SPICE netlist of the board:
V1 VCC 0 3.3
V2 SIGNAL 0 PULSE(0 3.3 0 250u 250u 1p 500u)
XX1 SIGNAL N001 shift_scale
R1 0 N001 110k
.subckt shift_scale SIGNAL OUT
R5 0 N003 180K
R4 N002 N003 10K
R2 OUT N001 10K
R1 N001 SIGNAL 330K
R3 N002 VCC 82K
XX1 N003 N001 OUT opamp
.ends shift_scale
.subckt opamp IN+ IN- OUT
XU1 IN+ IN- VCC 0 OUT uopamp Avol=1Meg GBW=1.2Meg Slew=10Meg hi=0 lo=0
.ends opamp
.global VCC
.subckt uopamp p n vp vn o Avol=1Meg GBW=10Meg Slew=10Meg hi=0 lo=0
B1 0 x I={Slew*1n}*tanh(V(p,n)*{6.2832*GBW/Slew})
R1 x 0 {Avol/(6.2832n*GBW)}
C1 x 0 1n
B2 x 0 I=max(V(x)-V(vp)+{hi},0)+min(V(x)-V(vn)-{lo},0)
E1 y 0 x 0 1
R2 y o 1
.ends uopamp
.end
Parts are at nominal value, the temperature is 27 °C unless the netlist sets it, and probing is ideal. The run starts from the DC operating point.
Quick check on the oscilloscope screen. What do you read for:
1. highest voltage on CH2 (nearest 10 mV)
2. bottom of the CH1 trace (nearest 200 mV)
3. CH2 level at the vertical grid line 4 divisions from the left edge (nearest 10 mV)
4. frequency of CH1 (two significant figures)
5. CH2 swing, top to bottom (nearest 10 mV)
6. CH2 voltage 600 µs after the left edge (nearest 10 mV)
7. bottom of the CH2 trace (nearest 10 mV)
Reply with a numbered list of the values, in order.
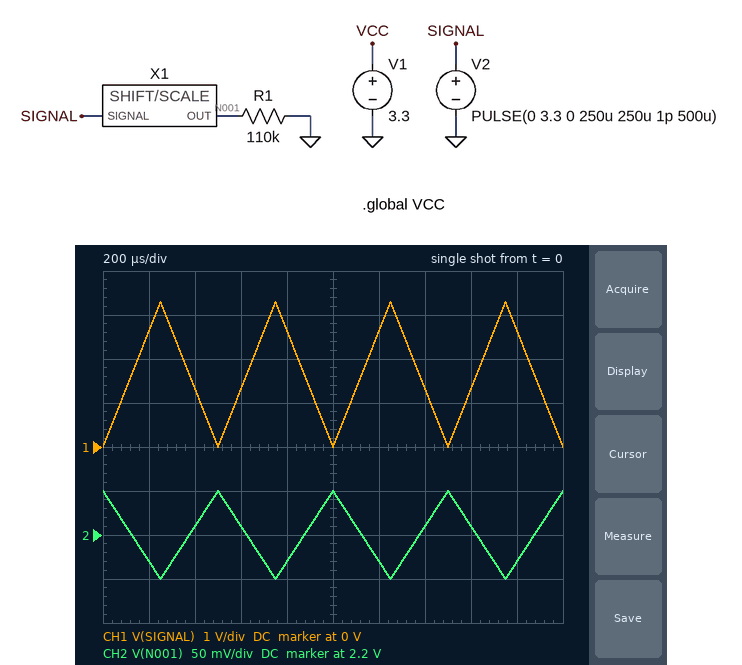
1. 2.25 V
2. 0 V
3. 2.17 V
4. 2.0 kHz
5. 100 mV
6. 2.21 V
7. 2.15 V
